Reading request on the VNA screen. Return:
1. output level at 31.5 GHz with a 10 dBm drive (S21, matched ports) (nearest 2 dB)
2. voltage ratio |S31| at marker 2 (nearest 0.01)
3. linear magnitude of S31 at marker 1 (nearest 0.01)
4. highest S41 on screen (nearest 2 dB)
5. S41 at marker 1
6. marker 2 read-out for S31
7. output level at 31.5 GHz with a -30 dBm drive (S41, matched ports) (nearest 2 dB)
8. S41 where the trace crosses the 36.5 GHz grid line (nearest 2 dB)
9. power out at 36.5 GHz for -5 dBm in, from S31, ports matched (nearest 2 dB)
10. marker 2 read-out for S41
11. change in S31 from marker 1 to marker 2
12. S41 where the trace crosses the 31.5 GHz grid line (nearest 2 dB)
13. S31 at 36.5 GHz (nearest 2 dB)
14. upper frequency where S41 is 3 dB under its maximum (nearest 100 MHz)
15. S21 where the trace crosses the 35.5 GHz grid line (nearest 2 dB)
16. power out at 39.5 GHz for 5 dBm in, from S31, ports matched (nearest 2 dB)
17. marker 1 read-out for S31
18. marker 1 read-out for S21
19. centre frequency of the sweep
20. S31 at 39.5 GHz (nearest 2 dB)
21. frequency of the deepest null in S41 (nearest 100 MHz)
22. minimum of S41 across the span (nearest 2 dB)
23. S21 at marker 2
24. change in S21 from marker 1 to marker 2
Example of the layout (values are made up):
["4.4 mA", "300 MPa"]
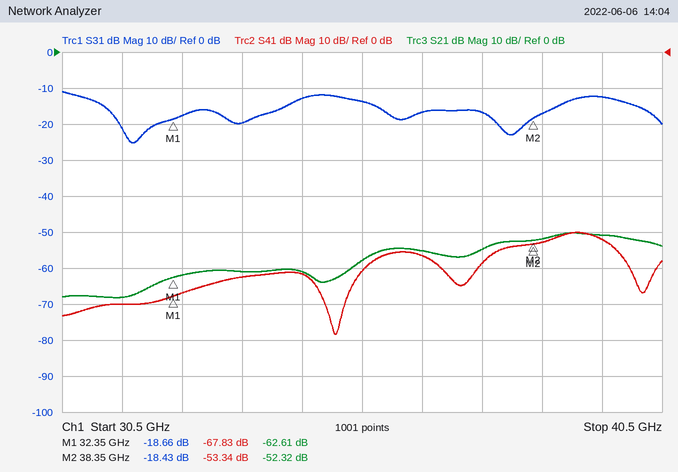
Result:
["-58 dBm", "0.12", "0.12", "-50 dB", "-67.83 dB", "-18.43 dB", "-100 dBm", "-56 dB", "-22 dBm", "-53.34 dB", "0.23 dB", "-70 dB", "-16 dB", "39.6 GHz", "-58 dB", "-8 dBm", "-18.66 dB", "-62.61 dB", "35.5 GHz", "-12 dB", "35.1 GHz", "-78 dB", "-52.32 dB", "10.29 dB"]
